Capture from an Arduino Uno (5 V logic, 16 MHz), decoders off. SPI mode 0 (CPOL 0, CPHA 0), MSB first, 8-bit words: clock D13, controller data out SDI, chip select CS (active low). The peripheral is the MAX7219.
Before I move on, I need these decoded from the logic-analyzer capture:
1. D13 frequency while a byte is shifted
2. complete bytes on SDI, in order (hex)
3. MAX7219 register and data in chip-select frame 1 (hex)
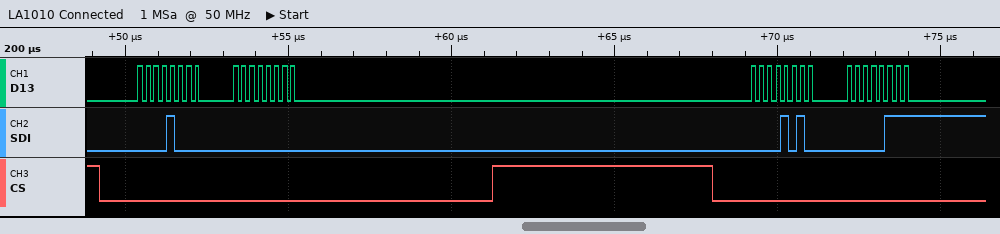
4 MHz
08 00 0A 07
register 0x8, data 0x00
